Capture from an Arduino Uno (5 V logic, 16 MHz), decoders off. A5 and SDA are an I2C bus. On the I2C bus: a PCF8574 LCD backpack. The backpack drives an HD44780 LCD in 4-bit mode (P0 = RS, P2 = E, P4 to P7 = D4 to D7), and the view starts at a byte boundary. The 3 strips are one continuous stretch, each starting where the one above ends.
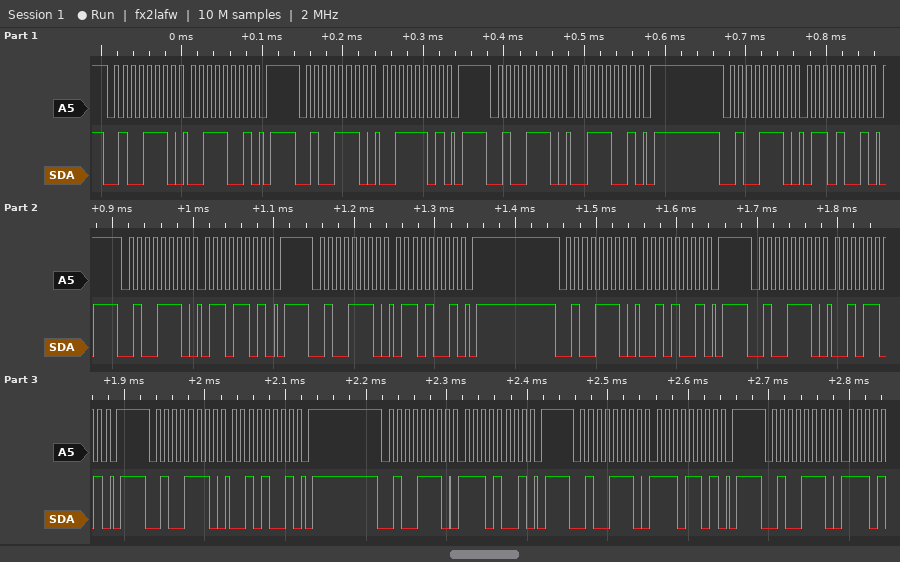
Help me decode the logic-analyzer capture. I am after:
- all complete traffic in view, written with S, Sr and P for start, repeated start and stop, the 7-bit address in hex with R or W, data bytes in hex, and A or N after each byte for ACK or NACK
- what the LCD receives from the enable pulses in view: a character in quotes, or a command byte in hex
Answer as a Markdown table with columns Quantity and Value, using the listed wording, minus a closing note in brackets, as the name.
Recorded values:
| Quantity | Value |
|---|---|
| all complete traffic in view, written with S, Sr and P for start, repeated start and stop, the 7-bit address in hex with R or W, data bytes in hex, and A or N after each byte for ACK or NACK | S 27W A 39 A P S 27W A 3D A P S 27W A 39 A P S 27W A 69 A P S 27W A 6D A P S 27W A 69 A P S 27W A 29 A P S 27W A 2D A P S 27W A 29 A P S 27W A E9 A P S 27W A ED A P S 27W A |
| what the LCD receives from the enable pulses in view: a character in quotes, or a command byte in hex | '6' |
